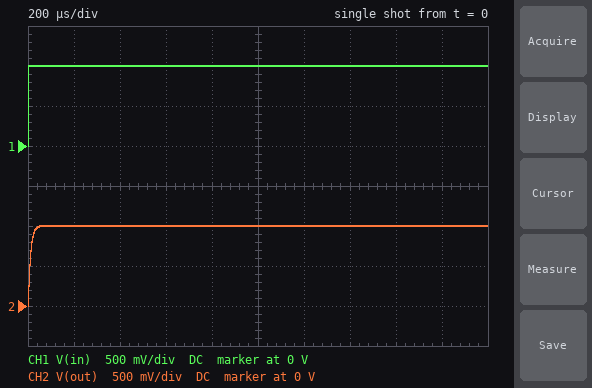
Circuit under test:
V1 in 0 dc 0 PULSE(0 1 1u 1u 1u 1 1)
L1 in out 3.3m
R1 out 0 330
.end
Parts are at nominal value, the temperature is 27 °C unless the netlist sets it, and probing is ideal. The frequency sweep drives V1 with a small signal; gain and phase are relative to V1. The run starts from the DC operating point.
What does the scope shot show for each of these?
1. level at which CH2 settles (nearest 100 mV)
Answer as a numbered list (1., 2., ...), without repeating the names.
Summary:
1. 1.0 V
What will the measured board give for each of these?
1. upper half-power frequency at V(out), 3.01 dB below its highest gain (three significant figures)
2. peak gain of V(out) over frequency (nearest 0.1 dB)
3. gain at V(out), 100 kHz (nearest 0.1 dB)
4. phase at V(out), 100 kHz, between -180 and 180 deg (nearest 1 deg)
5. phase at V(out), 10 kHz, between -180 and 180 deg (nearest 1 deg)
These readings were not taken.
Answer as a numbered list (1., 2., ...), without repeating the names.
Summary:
1. 15.9 kHz
2. 0 dB
3. -16.1 dB
4. -81 deg
5. -32 deg
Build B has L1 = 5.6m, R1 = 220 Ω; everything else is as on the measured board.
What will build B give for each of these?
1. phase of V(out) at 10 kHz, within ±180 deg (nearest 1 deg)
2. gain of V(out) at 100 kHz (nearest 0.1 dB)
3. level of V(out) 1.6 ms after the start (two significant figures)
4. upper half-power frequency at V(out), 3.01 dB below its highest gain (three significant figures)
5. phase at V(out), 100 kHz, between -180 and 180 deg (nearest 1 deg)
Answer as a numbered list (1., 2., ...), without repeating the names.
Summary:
1. -58 deg
2. -24.1 dB
3. 1.0 V
4. 6.25 kHz
5. -86 deg
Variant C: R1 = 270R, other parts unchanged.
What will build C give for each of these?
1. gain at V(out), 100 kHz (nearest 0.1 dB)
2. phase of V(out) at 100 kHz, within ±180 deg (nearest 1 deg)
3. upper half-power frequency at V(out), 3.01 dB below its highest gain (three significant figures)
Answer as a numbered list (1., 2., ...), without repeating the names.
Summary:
1. -17.8 dB
2. -83 deg
3. 13.0 kHz
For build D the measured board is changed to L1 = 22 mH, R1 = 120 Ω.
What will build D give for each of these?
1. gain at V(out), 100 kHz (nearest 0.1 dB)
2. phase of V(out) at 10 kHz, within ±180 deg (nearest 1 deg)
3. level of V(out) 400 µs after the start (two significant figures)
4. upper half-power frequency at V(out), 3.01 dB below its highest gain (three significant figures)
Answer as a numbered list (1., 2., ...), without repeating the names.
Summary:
1. -41.2 dB
2. -85 deg
3. 890 mV
4. 868 Hz
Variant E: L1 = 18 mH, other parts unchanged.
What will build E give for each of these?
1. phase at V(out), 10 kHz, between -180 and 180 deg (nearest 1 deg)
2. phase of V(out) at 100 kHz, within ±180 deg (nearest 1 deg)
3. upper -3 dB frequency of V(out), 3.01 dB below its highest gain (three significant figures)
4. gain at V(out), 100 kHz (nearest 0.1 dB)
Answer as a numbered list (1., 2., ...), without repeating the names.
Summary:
1. -74 deg
2. -88 deg
3. 2.92 kHz
4. -30.7 dB
